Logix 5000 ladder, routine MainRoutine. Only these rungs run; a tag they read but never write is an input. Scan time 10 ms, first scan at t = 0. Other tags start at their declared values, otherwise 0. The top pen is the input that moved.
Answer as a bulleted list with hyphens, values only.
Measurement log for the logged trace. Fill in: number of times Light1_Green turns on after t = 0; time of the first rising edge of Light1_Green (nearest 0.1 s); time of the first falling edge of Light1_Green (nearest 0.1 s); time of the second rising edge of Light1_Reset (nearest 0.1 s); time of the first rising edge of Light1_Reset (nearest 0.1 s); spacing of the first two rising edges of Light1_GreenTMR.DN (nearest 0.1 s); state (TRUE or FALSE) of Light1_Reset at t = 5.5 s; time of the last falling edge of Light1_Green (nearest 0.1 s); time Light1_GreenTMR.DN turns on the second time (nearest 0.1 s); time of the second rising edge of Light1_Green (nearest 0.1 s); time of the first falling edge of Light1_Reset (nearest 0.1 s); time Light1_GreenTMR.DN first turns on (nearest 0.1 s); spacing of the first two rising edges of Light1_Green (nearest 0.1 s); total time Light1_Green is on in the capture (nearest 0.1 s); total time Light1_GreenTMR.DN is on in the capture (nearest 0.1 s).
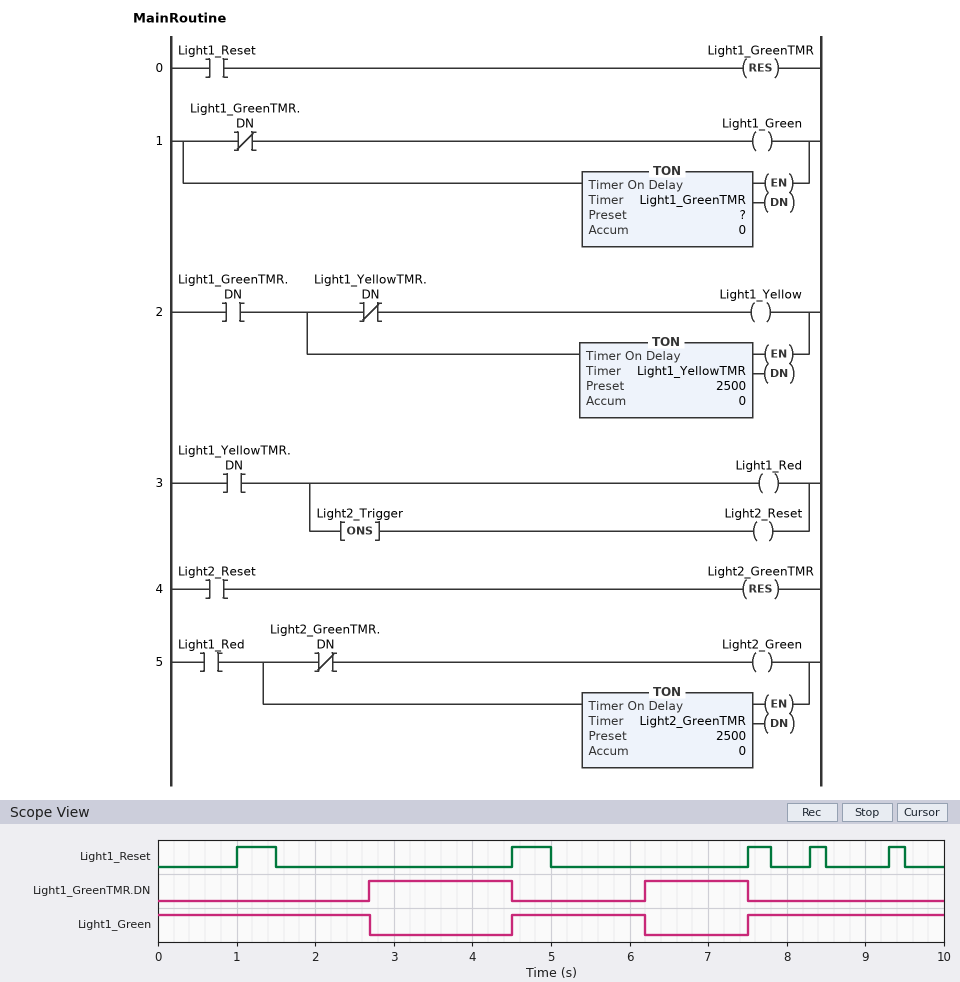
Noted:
- 2
- 4.5 s
- 2.7 s
- 4.5 s
- 1.0 s
- 3.5 s
- FALSE
- 6.2 s
- 6.2 s
- 7.5 s
- 1.5 s
- 2.7 s
- 3.0 s
- 6.9 s
- 3.1 s
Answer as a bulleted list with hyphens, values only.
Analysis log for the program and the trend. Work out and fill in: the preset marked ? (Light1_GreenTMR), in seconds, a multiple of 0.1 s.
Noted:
- 1.2 s
